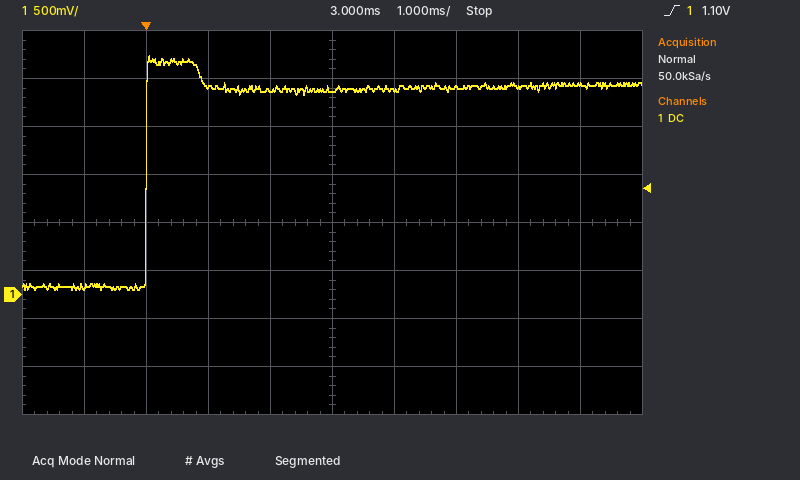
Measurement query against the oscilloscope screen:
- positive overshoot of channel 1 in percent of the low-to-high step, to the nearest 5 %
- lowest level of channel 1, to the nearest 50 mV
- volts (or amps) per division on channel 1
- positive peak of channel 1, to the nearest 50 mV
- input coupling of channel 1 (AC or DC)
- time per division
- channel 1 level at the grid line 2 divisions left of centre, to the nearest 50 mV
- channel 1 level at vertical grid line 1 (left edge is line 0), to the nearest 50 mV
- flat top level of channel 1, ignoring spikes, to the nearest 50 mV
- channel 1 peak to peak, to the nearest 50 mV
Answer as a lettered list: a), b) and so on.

a) 15 %
b) 50 mV
c) 500 mV
d) 2.50 V
e) DC
f) 1 ms
g) 2.15 V
h) 100 mV
i) 2.15 V
j) 2.45 V
